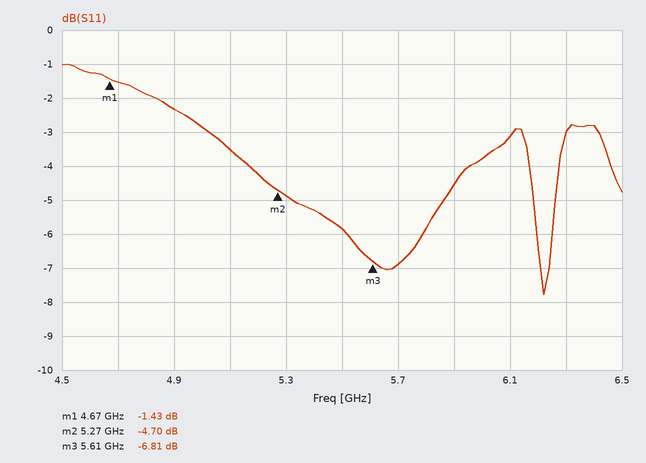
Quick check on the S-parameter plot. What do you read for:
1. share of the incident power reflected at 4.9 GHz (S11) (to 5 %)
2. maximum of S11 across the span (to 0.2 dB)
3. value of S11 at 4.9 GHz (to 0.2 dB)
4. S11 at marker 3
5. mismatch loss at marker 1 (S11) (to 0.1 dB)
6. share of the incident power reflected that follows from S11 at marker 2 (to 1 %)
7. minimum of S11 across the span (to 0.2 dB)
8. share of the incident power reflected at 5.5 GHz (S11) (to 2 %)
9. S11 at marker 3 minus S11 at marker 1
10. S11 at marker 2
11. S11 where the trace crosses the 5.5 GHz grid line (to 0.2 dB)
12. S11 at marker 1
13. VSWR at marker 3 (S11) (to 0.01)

60 %
-1.0 dB
-2.4 dB
-6.81 dB
5.5 dB
34 %
-7.8 dB
26 %
-5.38 dB
-4.70 dB
-5.8 dB
-1.43 dB
2.68
